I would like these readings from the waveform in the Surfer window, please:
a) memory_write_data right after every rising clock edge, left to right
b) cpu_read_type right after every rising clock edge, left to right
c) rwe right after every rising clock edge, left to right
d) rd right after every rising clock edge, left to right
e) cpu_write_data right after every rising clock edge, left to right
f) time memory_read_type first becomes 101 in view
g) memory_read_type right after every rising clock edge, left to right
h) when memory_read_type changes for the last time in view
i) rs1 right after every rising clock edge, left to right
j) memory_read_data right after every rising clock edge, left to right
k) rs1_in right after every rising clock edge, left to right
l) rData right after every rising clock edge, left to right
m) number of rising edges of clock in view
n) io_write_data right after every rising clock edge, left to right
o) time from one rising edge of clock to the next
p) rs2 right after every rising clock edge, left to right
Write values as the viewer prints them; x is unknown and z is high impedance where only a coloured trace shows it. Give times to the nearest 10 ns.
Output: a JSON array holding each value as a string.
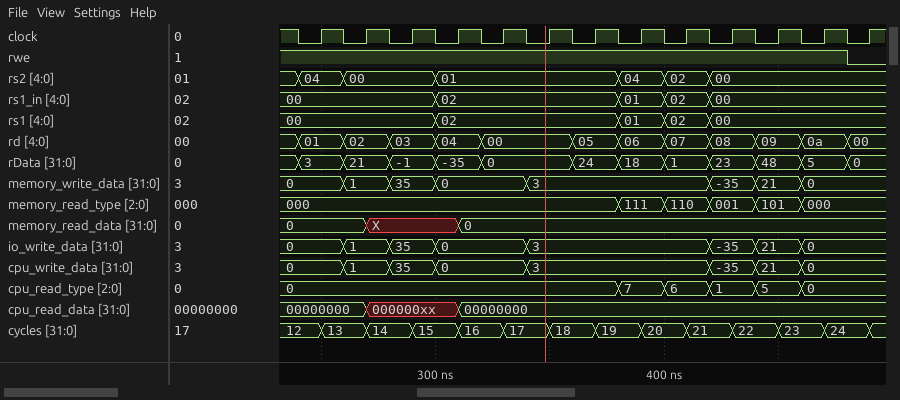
["0, 1, 35, 0, 0, 3, 3, 3, 3, -35, 21, 0, 0", "0, 0, 0, 0, 0, 0, 0, 7, 6, 1, 5, 0, 0", "1 1 1 1 1 1 1 1 1 1 1 1 0", "01, 02, 03, 04, 00, 00, 05, 06, 07, 08, 09, 0a, 00", "0, 1, 35, 0, 0, 3, 3, 3, 3, -35, 21, 0, 0", "440 ns", "000, 000, 000, 000, 000, 000, 000, 111, 110, 001, 101, 000, 000", "460 ns", "00, 00, 00, 02, 02, 02, 02, 01, 02, 00, 00, 00, 00", "0, X, X, 0, 0, 0, 0, 0, 0, 0, 0, 0, 0", "00, 00, 00, 02, 02, 02, 02, 01, 02, 00, 00, 00, 00", "3, 21, -1, -35, 0, 0, 24, 18, 1, 23, 48, 5, 0", "13", "0, 1, 35, 0, 0, 3, 3, 3, 3, -35, 21, 0, 0", "20 ns", "04, 00, 00, 01, 01, 01, 01, 04, 02, 00, 00, 00, 00"]
